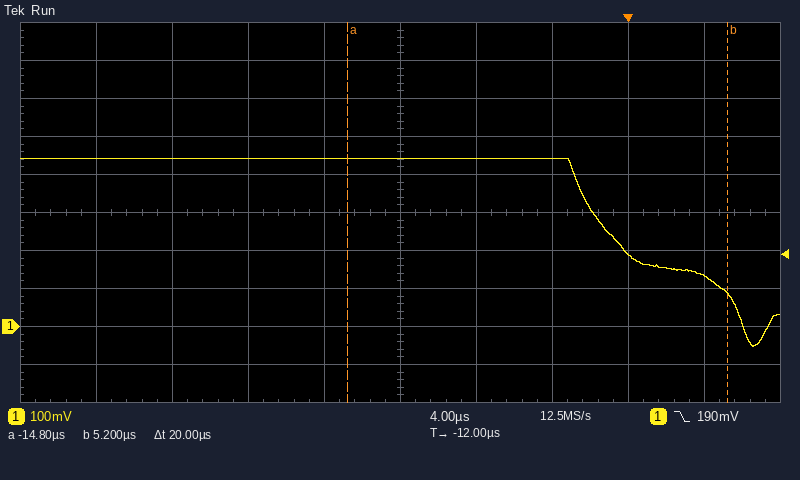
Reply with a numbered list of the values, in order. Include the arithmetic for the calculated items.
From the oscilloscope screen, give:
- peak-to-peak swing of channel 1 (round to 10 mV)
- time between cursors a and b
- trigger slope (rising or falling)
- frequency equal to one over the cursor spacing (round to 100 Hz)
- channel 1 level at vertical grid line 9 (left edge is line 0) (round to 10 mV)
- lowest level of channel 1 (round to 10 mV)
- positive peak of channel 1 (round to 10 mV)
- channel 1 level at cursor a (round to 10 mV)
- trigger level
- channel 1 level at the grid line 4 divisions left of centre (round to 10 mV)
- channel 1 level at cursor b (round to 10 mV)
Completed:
1. 440 mV − (-50 mV) = 490 mV
2. 20 µs
3. falling
4. 1 / 20 µs ≈ 50.0 kHz
5. 130 mV
6. -50 mV
7. 440 mV
8. 440 mV
9. 190 mV
10. 440 mV
11. 90 mV
